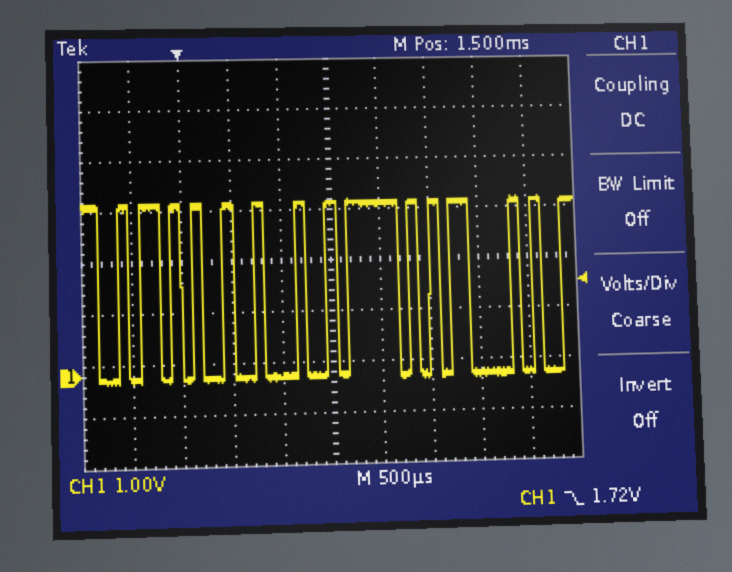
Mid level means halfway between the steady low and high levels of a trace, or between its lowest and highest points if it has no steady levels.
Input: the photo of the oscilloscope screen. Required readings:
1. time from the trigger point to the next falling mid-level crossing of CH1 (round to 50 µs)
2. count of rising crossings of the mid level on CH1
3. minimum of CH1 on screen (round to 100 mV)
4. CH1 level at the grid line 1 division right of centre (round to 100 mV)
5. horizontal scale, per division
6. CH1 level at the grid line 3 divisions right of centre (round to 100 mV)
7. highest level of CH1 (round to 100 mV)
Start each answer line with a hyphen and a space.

- 200 µs
- 15
- -200 mV
- 3.3 V
- 500 µs
- -100 mV
- 3.4 V
